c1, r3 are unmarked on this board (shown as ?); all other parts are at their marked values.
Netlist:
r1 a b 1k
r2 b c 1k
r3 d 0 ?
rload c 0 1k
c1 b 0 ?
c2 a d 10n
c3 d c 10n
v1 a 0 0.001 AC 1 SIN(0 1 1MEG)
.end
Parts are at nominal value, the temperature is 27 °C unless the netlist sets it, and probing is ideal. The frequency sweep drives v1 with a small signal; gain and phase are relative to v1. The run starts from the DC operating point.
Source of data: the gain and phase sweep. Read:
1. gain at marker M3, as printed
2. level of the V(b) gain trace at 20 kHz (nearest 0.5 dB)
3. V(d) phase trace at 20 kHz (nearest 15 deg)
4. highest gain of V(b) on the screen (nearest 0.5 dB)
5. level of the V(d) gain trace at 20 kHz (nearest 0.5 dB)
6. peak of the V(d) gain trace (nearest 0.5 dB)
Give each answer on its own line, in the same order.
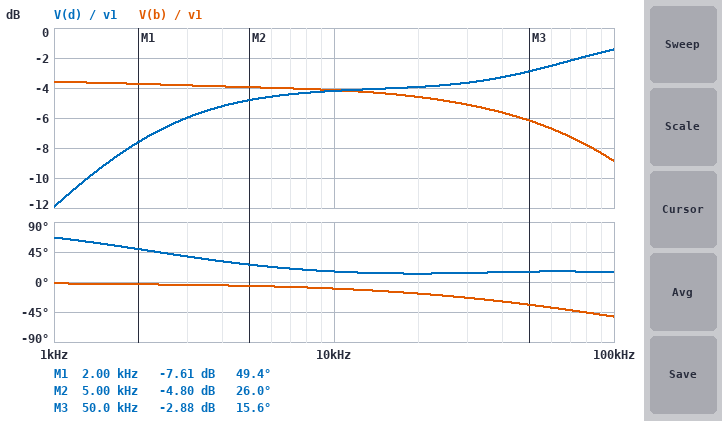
-2.88 dB
-4.5 dB
15 deg
-3.5 dB
-4.0 dB
-1.5 dB
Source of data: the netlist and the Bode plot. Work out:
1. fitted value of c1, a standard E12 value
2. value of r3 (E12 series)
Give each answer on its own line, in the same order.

6.8 nF
3.3 kΩ
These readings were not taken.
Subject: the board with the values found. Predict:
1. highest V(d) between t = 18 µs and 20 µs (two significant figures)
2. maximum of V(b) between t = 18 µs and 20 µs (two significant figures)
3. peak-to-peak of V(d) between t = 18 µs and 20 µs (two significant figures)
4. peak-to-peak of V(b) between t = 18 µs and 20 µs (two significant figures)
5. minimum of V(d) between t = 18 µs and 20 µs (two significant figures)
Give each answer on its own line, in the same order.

1.0 V
47 mV
2.0 V
93 mV
-1.0 V
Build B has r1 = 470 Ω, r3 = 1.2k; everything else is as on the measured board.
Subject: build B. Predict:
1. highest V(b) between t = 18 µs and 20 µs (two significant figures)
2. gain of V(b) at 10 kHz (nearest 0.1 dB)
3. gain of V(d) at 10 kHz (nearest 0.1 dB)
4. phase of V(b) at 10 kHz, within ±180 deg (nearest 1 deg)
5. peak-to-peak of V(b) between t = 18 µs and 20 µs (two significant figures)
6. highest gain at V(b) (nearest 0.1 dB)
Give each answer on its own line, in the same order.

73 mV
-2.3 dB
-5.4 dB
-8 deg
150 mV
-1.8 dB
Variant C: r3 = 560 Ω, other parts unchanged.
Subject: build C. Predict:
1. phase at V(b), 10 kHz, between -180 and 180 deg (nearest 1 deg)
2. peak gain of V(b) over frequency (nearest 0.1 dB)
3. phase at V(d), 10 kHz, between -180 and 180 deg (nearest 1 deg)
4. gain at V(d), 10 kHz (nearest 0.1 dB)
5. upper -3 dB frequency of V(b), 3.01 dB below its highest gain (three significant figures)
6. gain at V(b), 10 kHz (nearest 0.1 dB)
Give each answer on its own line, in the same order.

-15 deg
-3.5 dB
52 deg
-9.4 dB
33.1 kHz
-4.8 dB
